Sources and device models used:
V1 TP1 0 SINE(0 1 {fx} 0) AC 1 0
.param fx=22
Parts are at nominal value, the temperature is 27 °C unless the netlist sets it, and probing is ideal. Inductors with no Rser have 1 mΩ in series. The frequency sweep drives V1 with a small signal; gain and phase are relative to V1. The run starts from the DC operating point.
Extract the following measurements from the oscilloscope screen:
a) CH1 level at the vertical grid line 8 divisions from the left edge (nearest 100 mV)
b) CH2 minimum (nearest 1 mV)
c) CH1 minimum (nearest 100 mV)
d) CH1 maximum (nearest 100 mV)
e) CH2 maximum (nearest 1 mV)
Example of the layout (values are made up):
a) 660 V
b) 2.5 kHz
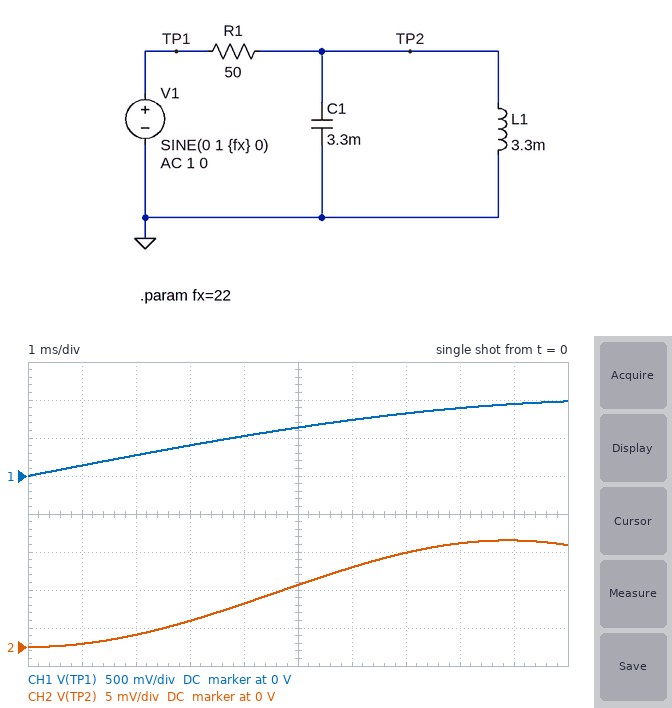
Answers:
a) 900 mV
b) 0 V
c) 0 V
d) 1.0 V
e) 14 mV
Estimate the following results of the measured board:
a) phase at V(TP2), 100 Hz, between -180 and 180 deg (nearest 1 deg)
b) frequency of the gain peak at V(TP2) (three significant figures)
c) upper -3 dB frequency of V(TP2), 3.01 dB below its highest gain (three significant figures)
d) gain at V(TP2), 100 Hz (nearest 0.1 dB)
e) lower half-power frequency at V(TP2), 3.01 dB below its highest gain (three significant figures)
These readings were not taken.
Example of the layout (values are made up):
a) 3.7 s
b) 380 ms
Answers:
a) -89 deg
b) 48.2 Hz
c) 48.7 Hz
d) -38.0 dB
e) 47.7 Hz
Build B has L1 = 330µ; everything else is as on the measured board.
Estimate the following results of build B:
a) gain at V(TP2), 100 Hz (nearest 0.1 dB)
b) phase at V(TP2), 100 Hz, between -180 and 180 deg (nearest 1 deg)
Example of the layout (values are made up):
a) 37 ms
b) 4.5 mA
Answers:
a) -42.8 dB
b) 89 deg
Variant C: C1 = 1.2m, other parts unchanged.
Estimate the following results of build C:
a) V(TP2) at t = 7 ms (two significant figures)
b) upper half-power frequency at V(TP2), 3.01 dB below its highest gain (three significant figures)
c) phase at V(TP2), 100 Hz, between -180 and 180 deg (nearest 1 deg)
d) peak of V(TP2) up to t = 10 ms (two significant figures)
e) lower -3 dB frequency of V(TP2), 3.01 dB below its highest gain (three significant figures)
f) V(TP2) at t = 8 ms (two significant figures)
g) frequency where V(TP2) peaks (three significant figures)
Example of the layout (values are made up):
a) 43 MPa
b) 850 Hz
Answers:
a) 14 mV
b) 81.3 Hz
c) -86 deg
d) 16 mV
e) 78.6 Hz
f) 11 mV
g) 80.0 Hz
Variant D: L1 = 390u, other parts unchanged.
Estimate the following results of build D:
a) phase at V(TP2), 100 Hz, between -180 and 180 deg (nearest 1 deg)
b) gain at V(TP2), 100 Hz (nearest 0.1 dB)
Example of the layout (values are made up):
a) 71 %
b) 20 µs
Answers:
a) 89 deg
b) -40.0 dB
